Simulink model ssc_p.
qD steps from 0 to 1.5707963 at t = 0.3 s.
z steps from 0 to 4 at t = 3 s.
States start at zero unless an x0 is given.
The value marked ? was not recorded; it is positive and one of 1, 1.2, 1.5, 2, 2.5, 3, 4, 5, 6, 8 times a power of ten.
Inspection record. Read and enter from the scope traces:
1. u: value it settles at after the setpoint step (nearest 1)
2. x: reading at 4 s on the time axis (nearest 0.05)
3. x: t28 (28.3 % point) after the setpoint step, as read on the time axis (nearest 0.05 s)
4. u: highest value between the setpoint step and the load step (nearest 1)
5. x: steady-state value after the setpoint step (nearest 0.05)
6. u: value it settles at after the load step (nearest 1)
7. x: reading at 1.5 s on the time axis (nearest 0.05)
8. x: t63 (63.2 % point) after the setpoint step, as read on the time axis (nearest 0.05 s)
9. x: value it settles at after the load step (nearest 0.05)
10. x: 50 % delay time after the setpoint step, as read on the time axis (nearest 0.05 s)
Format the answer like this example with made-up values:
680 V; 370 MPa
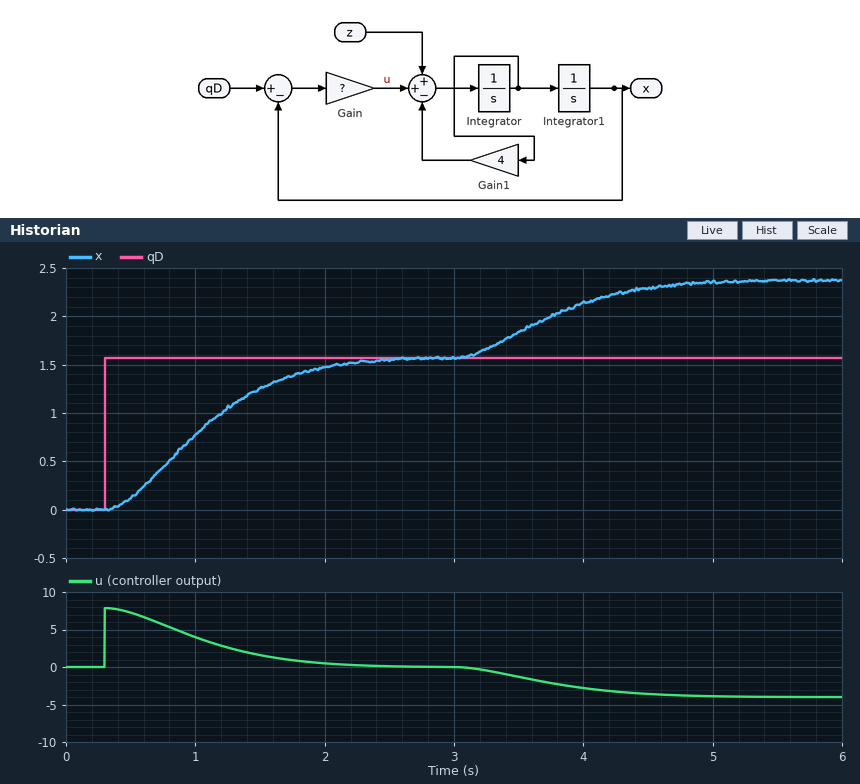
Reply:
0; 2.15; 0.75 s; 8; 1.55; -4; 1.25; 1.20 s; 2.35; 1.00 s
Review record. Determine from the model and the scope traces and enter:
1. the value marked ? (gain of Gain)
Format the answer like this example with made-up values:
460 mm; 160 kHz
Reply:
5
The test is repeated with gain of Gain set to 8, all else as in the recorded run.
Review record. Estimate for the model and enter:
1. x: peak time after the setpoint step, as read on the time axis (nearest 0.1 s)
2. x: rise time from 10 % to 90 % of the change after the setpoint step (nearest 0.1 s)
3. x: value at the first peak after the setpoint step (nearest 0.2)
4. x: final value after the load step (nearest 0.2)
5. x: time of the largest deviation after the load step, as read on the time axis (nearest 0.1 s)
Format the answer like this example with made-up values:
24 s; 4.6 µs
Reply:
1.9 s; 0.8 s; 1.6; 2.0; 4.6 s
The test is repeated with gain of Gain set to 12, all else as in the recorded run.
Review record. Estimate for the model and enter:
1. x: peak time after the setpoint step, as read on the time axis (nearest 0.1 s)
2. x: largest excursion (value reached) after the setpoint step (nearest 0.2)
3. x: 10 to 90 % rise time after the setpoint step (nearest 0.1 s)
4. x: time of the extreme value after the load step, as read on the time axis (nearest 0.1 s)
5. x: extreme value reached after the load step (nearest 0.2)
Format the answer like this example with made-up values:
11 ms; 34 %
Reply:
1.4 s; 1.8; 0.5 s; 4.1 s; 2.0
